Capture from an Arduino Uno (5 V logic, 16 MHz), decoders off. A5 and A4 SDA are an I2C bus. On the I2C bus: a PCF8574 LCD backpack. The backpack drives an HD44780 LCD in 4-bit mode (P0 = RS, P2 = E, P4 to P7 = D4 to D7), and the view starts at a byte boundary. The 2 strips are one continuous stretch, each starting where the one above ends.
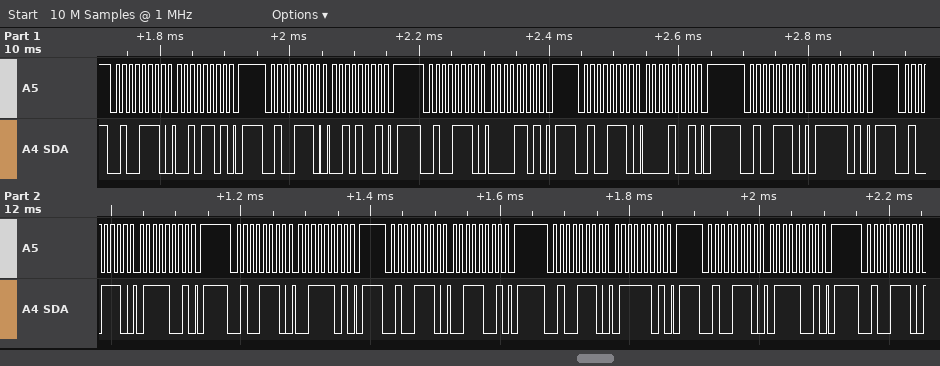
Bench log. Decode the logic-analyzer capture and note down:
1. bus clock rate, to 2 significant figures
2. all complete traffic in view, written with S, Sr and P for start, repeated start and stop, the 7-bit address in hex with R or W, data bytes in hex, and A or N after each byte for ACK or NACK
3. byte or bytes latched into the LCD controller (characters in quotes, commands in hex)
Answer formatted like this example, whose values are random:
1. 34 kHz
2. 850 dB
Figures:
1. 100 kHz
2. S 27W A 2D A P S 27W A 29 A P S 27W A 0D A P S 27W A 09 A P S 27W A 7D A P S 27W A 79 A P S 27W A 3D A P S 27W A 39 A P S 27W A 7D A P S 27W A 79 A P S 27W A
3. ' ' 's'
